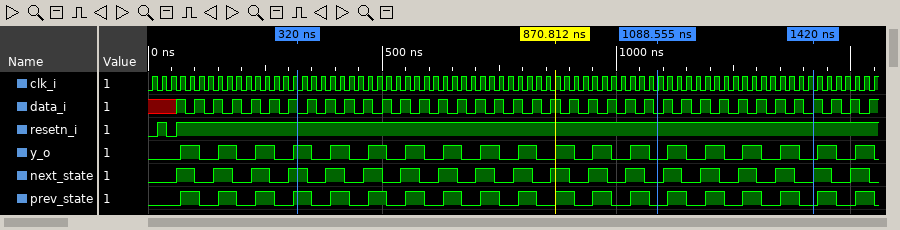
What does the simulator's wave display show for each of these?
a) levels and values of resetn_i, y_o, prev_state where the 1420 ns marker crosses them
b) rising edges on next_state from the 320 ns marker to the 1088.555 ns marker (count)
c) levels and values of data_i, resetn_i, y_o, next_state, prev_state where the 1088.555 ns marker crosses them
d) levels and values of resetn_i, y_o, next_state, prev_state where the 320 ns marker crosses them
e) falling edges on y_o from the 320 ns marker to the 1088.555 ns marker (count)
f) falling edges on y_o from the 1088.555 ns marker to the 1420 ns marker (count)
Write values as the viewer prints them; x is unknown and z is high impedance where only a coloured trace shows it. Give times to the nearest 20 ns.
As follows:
resetn_i=1, y_o=0, prev_state=0
9
data_i=0, resetn_i=1, y_o=0, next_state=0, prev_state=0
resetn_i=1, y_o=1, next_state=1, prev_state=1
10
4
